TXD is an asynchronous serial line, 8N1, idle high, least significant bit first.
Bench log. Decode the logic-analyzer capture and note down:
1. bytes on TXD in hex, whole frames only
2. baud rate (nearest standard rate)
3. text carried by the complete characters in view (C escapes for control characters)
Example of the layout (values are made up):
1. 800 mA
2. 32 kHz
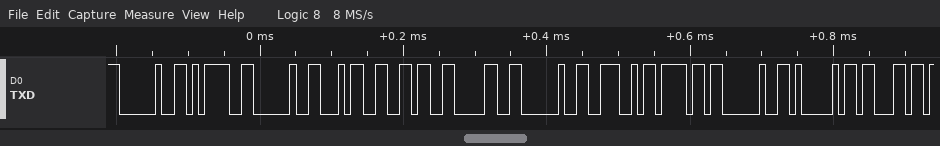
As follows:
1. 0x20 0x3D 0x20 0x34 0x36 0x30 0x20 0x4E 0x6F 0x20 0x41 0x63
2. 115200 baud
3. " = 460 No Ac"
